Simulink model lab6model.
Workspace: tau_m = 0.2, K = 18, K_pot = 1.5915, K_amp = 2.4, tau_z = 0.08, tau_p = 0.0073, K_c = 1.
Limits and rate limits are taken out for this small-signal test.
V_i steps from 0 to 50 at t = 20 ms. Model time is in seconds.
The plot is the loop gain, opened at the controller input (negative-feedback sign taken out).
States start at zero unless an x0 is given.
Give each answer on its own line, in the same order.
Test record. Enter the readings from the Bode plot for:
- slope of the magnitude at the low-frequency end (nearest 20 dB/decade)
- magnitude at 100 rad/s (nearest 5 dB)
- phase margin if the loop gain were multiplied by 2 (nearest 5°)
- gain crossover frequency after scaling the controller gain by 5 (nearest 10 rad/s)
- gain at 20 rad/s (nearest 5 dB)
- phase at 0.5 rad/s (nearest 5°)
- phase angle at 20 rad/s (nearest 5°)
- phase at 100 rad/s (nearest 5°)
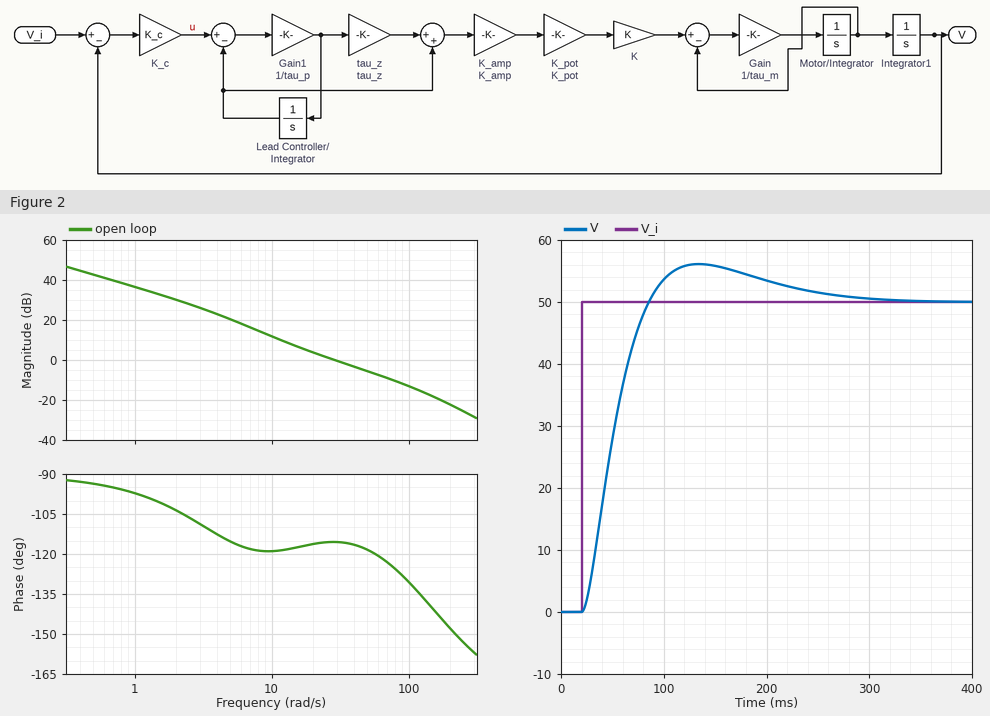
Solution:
-20 dB/decade
-15 dB
60°
110 rad/s
5 dB
-95°
-115°
-130°
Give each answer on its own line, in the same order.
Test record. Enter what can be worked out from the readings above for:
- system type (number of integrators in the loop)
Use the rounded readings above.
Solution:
1
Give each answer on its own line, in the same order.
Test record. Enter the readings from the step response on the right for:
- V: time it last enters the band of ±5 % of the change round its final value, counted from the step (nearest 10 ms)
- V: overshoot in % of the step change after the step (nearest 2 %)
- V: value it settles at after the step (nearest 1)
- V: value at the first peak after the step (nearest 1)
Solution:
200 ms
12 %
50
56
